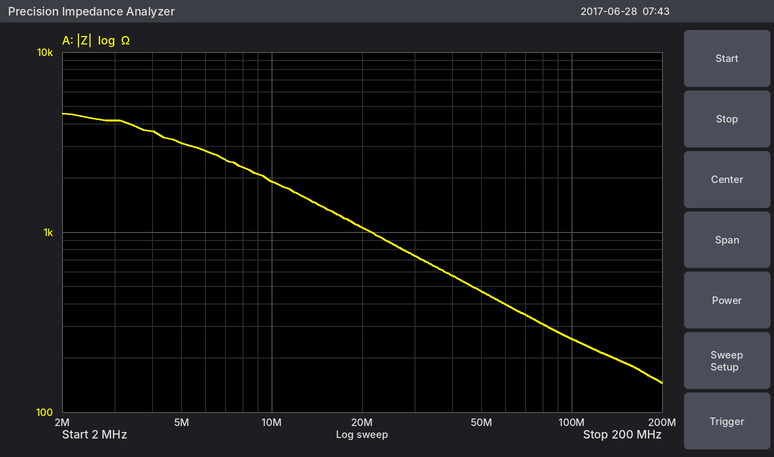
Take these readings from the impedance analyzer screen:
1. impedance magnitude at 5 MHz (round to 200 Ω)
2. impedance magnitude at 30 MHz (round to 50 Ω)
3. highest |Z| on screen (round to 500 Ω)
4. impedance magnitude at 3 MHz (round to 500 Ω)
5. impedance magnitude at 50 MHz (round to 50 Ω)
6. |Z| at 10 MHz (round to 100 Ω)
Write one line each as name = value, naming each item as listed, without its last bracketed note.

impedance magnitude at 5 MHz = 3.2 kΩ
impedance magnitude at 30 MHz = 750 Ω
highest |Z| on screen = 4.5 kΩ
impedance magnitude at 3 MHz = 4.0 kΩ
impedance magnitude at 50 MHz = 450 Ω
|Z| at 10 MHz = 1.9 kΩ
